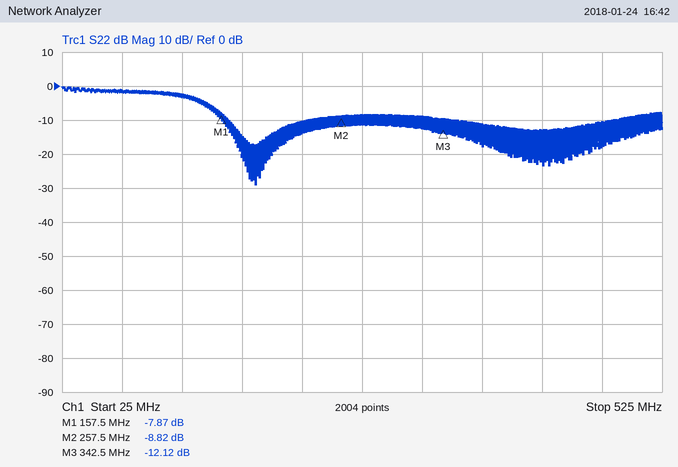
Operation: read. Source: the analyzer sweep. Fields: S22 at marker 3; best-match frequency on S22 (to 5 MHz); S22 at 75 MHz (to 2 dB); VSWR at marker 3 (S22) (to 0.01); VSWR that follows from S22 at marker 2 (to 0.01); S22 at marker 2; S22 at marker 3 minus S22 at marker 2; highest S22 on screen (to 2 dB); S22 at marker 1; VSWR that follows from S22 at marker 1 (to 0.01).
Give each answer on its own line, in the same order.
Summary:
-12.12 dB
185 MHz
-2 dB
1.66
2.14
-8.82 dB
-3.30 dB
0 dB
-7.87 dB
2.36
